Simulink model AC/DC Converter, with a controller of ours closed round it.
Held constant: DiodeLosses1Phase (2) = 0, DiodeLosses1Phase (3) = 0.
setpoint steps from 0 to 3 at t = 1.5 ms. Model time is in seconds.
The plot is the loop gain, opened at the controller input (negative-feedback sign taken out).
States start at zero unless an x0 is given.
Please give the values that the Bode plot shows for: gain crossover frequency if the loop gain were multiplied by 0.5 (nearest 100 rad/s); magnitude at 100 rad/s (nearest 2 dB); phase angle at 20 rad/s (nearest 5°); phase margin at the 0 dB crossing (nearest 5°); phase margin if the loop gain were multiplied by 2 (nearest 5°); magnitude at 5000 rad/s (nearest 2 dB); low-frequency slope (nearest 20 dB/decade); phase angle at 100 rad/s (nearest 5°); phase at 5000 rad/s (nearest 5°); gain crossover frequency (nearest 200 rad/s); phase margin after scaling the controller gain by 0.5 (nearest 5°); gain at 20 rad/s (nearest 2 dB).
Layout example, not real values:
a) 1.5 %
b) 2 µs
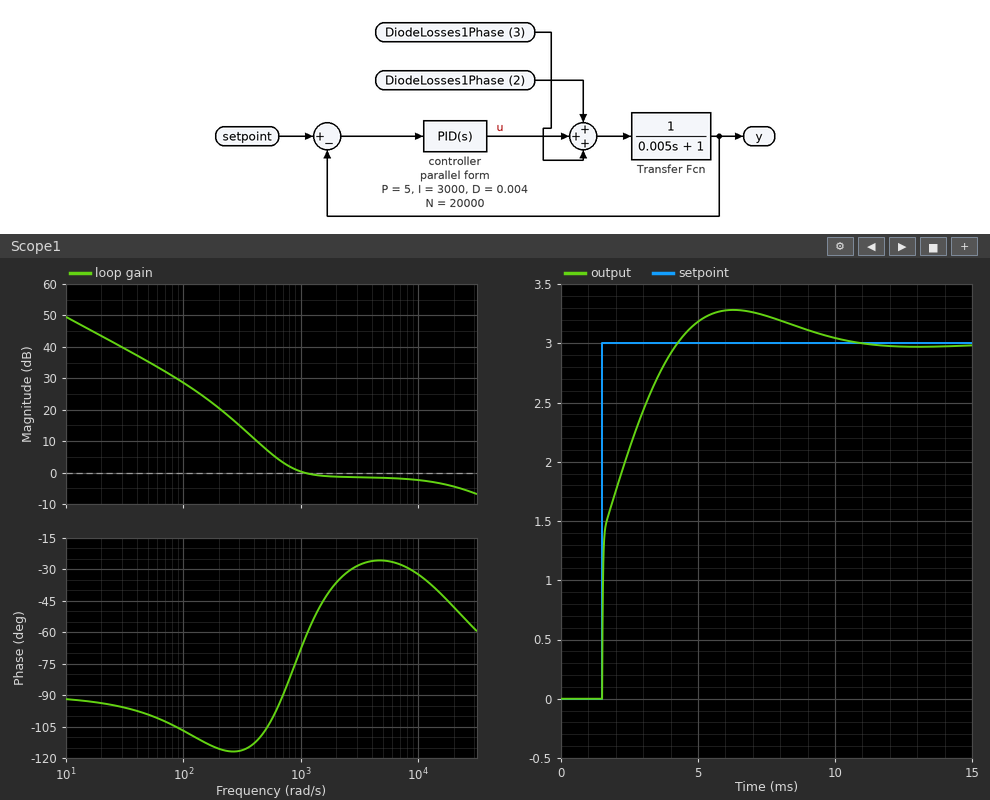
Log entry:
a) 600 rad/s
b) 28 dB
c) -95°
d) 115°
e) 125°
f) -2 dB
g) -20 dB/decade
h) -105°
i) -25°
j) 1000 rad/s
k) 80°
l) 44 dB
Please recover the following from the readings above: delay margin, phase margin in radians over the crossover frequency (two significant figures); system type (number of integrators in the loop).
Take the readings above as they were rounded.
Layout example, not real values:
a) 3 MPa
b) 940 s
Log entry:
a) 0.0020 s
b) 1
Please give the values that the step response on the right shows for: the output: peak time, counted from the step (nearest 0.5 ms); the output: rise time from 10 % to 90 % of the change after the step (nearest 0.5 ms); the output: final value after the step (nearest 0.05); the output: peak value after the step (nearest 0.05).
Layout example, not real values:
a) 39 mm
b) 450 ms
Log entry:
a) 5.0 ms
b) 2.0 ms
c) 3.00
d) 3.30
